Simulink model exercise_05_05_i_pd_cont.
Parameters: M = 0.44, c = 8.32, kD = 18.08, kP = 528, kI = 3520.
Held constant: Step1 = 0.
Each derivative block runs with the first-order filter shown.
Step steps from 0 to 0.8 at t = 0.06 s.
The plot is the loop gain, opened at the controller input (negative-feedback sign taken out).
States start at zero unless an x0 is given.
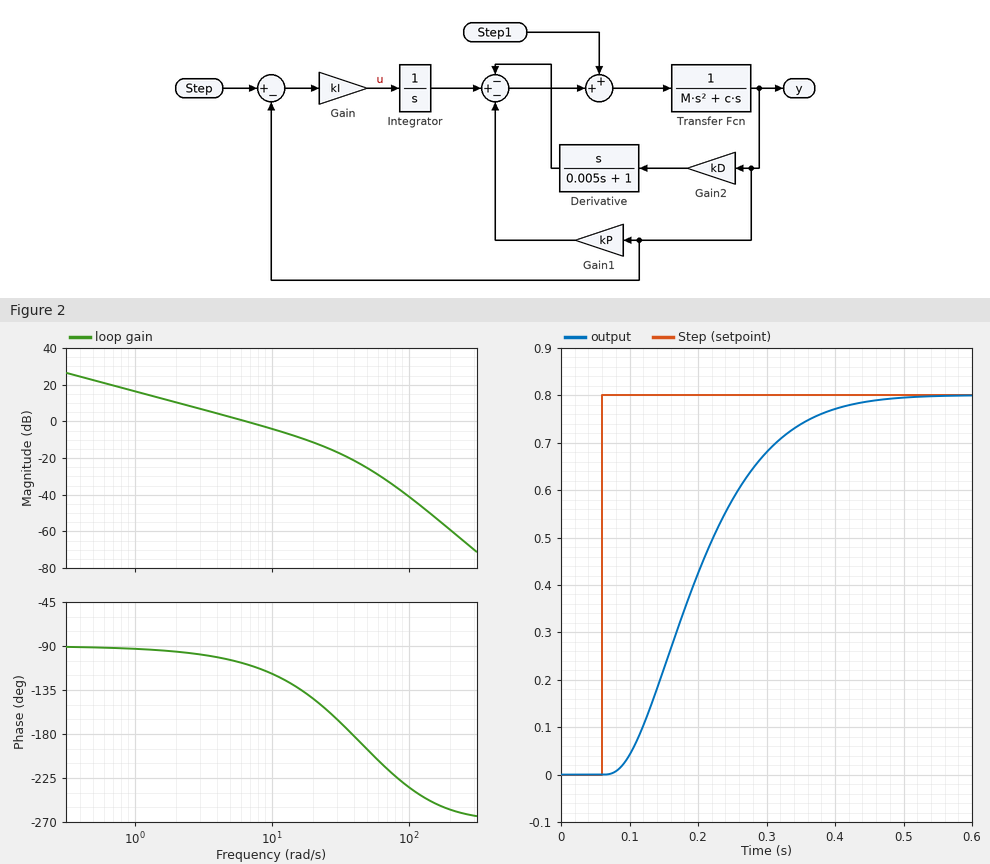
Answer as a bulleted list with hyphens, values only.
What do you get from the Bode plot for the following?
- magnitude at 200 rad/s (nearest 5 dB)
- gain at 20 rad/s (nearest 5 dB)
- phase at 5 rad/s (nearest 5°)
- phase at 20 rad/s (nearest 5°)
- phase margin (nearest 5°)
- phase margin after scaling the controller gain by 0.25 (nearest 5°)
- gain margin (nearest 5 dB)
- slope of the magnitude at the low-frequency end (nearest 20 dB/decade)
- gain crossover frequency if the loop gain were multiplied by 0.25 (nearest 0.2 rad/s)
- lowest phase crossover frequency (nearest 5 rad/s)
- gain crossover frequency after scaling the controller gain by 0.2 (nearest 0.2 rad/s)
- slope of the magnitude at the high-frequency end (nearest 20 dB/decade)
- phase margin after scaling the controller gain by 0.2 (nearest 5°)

- -60 dB
- -10 dB
- -105°
- -145°
- 70°
- 85°
- 20 dB
- -20 dB/decade
- 1.6 rad/s
- 40 rad/s
- 1.4 rad/s
- -60 dB/decade
- 85°
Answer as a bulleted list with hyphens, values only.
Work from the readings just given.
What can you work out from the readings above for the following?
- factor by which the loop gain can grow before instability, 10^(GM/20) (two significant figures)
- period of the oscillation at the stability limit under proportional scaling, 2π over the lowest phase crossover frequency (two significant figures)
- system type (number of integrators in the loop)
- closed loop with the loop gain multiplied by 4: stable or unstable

- 10
- 0.16 s
- 1
- stable
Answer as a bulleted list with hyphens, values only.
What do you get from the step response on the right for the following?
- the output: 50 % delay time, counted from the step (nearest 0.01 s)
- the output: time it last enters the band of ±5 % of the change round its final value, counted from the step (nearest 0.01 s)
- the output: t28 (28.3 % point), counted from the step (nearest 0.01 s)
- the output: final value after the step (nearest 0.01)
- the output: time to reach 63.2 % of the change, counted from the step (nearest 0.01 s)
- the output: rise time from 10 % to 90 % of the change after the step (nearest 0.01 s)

- 0.13 s
- 0.32 s
- 0.09 s
- 0.80
- 0.16 s
- 0.22 s
